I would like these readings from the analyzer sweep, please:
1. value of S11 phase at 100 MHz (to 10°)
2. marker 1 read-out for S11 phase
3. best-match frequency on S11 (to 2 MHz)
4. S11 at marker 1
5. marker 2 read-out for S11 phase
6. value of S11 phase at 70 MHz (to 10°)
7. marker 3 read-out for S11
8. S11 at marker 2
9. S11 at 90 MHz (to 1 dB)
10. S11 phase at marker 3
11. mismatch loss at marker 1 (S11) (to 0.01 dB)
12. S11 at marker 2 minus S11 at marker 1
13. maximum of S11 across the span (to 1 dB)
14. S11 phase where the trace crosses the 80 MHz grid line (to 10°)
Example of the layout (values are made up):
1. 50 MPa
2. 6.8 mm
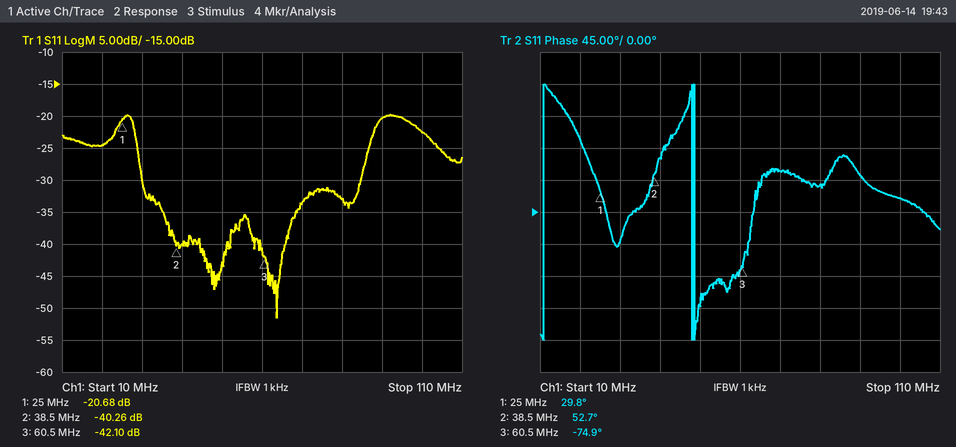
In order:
1. 20°
2. 29.8°
3. 64 MHz
4. -20.68 dB
5. 52.7°
6. 60°
7. -42.10 dB
8. -40.26 dB
9. -20 dB
10. -74.9°
11. 0.04 dB
12. -19.58 dB
13. -20 dB
14. 40°
